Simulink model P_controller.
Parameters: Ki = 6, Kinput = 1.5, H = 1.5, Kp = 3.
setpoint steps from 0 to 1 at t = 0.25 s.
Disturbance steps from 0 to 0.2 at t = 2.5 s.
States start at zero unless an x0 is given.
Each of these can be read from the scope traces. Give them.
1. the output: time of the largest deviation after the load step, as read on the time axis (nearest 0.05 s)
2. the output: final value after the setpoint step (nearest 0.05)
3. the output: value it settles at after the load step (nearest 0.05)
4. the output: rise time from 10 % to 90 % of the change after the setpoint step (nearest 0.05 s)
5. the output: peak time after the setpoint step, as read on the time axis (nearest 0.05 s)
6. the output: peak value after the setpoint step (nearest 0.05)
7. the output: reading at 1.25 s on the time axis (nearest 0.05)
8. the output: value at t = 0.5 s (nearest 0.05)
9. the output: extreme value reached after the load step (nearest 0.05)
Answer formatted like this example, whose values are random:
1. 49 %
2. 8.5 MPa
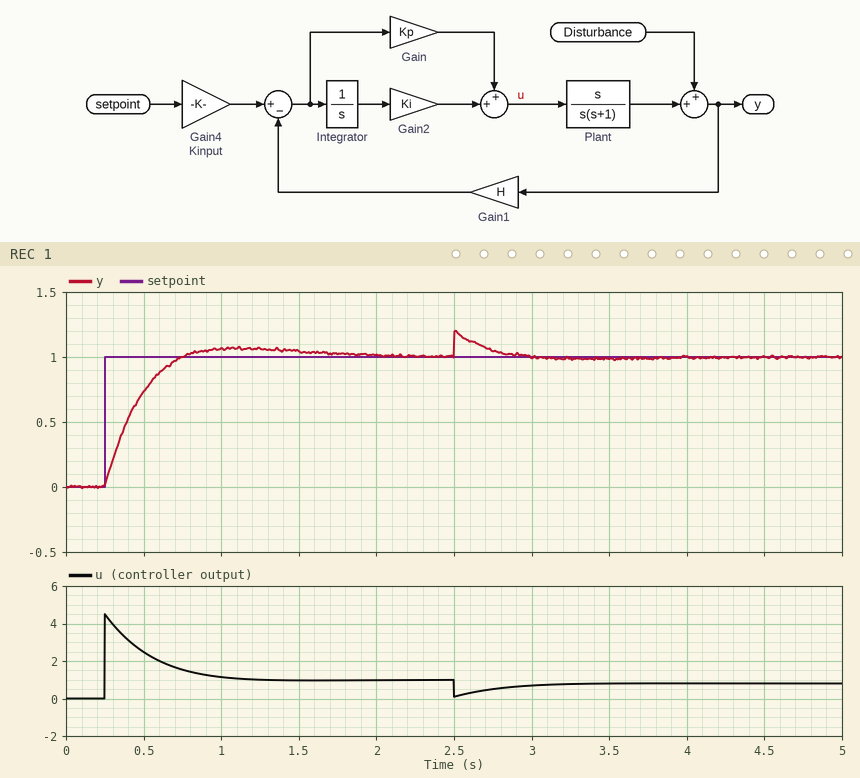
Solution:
1. 2.50 s
2. 1.00
3. 1.00
4. 0.35 s
5. 1.10 s
6. 1.05
7. 1.05
8. 0.75
9. 1.20
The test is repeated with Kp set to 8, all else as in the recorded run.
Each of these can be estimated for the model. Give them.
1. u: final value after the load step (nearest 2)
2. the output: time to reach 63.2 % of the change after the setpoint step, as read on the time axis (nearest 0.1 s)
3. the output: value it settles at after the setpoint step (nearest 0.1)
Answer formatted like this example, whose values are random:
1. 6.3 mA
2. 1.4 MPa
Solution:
1. 0
2. 0.3 s
3. 1.0
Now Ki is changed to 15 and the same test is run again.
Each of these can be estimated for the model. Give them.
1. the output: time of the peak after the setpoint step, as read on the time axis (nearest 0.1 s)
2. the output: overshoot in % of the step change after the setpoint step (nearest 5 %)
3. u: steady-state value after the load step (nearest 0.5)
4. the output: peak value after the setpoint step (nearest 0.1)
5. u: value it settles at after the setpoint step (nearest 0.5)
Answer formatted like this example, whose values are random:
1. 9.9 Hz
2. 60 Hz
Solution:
1. 0.8 s
2. 20 %
3. 1.0
4. 1.2
5. 1.0
